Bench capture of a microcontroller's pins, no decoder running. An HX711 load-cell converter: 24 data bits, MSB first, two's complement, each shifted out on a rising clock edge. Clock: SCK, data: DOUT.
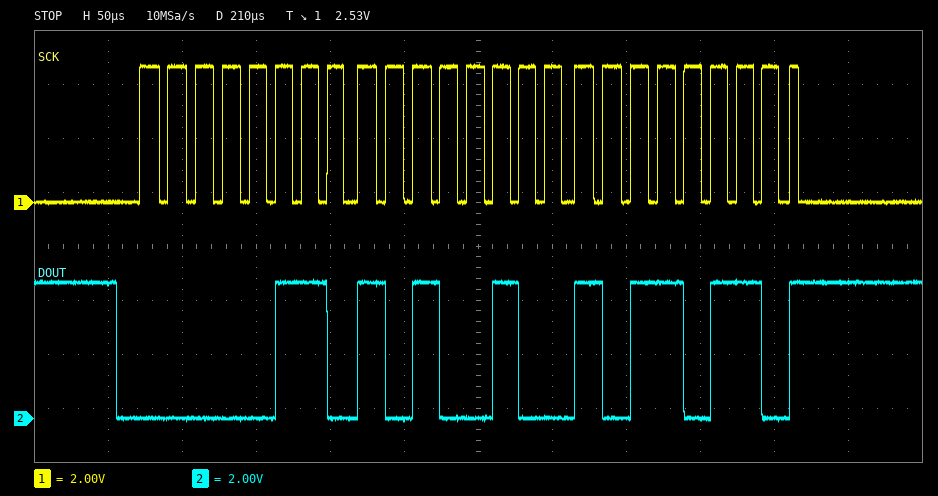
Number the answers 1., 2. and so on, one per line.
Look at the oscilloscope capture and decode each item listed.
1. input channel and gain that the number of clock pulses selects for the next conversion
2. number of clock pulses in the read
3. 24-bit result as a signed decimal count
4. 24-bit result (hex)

1. channel A, gain 128
2. 25
3. 435382
4. 0x06A4B6
